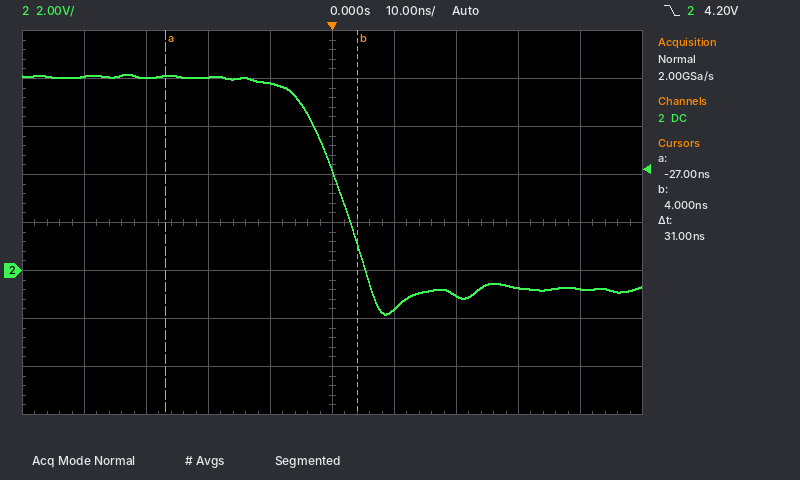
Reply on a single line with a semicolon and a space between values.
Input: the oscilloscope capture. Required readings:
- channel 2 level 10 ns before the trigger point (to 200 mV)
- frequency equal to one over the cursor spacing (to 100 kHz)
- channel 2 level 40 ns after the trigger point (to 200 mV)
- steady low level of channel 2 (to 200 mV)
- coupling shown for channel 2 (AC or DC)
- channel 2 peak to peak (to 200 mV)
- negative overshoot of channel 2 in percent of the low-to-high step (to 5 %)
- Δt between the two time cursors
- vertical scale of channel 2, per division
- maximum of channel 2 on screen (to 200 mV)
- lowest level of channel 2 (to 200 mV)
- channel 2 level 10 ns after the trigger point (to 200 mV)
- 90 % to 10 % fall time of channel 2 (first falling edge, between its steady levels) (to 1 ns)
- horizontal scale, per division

7.8 V; 32.3 MHz; -800 mV; -800 mV; DC; 10.0 V; 10 %; 31 ns; 2 V; 8.2 V; -1.8 V; -1.6 V; 11 ns; 10 ns
